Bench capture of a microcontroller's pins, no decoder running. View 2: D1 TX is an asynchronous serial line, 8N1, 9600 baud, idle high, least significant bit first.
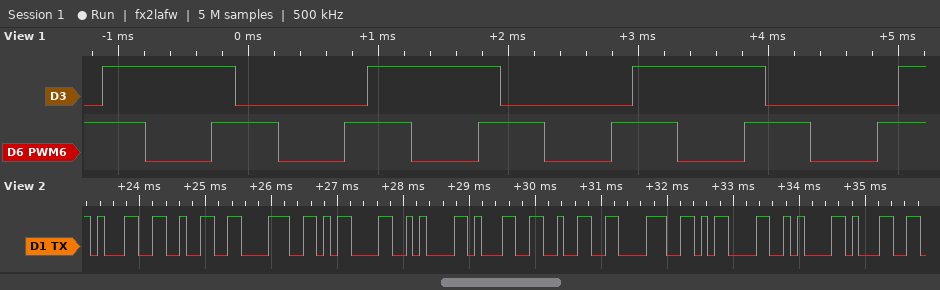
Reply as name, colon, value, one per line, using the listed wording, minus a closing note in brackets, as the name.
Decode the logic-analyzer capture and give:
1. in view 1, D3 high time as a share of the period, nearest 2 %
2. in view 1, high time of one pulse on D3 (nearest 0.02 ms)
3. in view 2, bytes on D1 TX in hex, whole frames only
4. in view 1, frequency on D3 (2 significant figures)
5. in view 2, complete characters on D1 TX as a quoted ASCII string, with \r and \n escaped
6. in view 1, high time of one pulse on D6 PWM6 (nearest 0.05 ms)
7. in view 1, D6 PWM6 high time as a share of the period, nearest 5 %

in view 1, D3 high time as a share of the period, nearest 2 %: 50 %
in view 1, high time of one pulse on D3: 1.02 ms
in view 2, bytes on D1 TX in hex, whole frames only: 0x31 0x32 0x38 0x0D 0x0A 0x31 0x32 0x38 0x0D 0x0A 0x31
in view 1, frequency on D3: 490 Hz
in view 2, complete characters on D1 TX as a quoted ASCII string, with \r and \n escaped: "128\r\n128\r\n1"
in view 1, high time of one pulse on D6 PWM6: 0.50 ms
in view 1, D6 PWM6 high time as a share of the period, nearest 5 %: 50 %
